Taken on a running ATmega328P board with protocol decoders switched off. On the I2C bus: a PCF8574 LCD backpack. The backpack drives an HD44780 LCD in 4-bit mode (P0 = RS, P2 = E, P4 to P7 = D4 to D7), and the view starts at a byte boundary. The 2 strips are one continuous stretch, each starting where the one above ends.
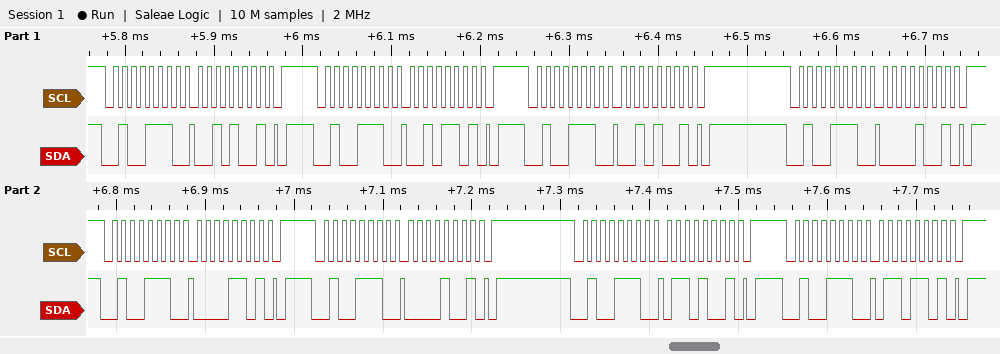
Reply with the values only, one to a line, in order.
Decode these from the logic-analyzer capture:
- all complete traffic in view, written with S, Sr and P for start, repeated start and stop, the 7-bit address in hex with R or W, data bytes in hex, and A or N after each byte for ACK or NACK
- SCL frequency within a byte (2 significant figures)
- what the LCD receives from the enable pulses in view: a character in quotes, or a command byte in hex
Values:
S 27W A 29 A P S 27W A 2D A P S 27W A 29 A P S 27W A 09 A P S 27W A 0D A P S 27W A 09 A P S 27W A 69 A P S 27W A 6D A P
100 kHz
' '
